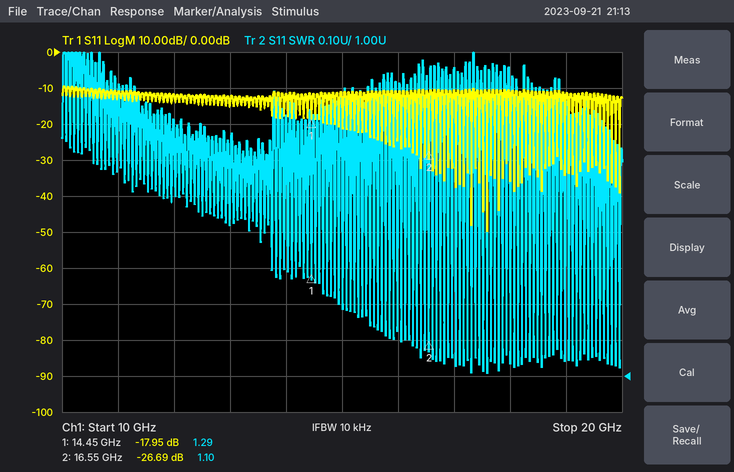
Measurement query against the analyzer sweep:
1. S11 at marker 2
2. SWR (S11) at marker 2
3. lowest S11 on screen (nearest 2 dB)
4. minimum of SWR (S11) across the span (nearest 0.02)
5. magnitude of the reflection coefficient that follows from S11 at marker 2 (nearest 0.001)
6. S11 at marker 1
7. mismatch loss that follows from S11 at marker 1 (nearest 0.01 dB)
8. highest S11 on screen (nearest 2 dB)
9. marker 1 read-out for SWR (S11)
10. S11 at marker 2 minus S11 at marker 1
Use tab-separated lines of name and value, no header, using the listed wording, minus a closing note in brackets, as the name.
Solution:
S11 at marker 2	-26.69 dB
SWR (S11) at marker 2	1.10
lowest S11 on screen	-50 dB
minimum of SWR (S11) across the span	1.00
magnitude of the reflection coefficient that follows from S11 at marker 2	0.046
S11 at marker 1	-17.95 dB
mismatch loss that follows from S11 at marker 1	0.07 dB
highest S11 on screen	-10 dB
marker 1 read-out for SWR	1.29
S11 at marker 2 minus S11 at marker 1	-8.74 dB
